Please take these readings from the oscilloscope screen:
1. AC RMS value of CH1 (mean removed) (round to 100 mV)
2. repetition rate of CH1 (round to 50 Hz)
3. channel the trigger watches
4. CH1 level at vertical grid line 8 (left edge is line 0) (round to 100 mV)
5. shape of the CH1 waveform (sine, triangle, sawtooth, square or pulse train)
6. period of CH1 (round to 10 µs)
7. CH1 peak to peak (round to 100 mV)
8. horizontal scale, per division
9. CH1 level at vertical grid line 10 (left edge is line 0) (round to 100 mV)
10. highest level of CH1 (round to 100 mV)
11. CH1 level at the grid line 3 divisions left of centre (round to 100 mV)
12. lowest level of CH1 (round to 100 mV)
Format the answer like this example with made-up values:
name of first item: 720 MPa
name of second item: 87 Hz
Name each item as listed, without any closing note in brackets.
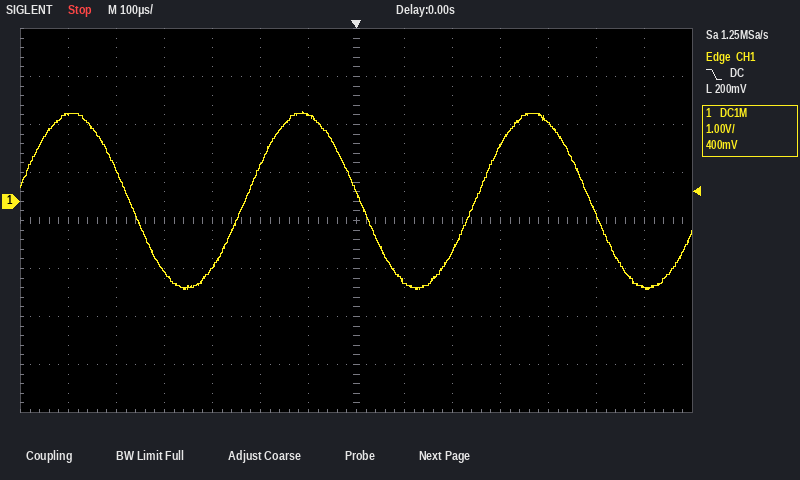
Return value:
AC RMS value of CH1 (mean removed): 1.3 V
repetition rate of CH1: 2.10 kHz
channel the trigger watches: CH1
CH1 level at vertical grid line 8 (left edge is line 0): -1.7 V
shape of the CH1 waveform: sine
period of CH1: 480 µs
CH1 peak to peak: 3.7 V
horizontal scale, per division: 100 µs
CH1 level at vertical grid line 10 (left edge is line 0): 1.2 V
highest level of CH1: 1.9 V
CH1 level at the grid line 3 divisions left of centre: -1.4 V
lowest level of CH1: -1.8 V
